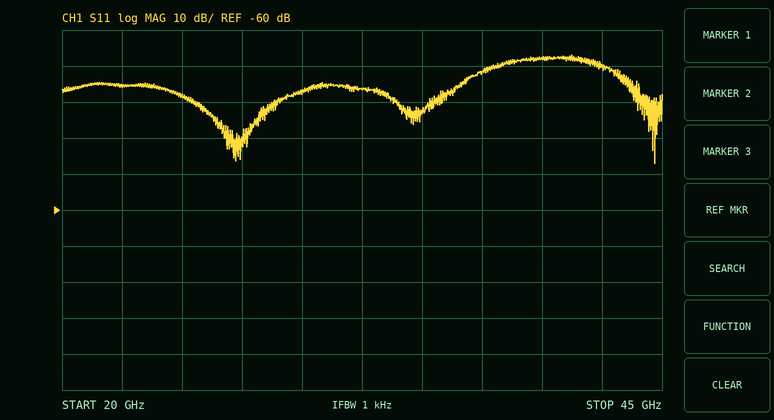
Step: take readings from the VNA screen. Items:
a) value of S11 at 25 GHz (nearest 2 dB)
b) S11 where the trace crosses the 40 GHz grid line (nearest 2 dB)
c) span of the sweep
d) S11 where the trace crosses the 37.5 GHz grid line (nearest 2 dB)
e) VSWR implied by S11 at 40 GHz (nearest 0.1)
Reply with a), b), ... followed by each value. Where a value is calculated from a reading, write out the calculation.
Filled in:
a) -28 dB
b) -18 dB
c) 25 GHz
d) -22 dB
e) |Γ| = 10^(-18/20) = 0.1259; VSWR = (1 + 0.1259)/(1 − 0.1259) ≈ 1.3
